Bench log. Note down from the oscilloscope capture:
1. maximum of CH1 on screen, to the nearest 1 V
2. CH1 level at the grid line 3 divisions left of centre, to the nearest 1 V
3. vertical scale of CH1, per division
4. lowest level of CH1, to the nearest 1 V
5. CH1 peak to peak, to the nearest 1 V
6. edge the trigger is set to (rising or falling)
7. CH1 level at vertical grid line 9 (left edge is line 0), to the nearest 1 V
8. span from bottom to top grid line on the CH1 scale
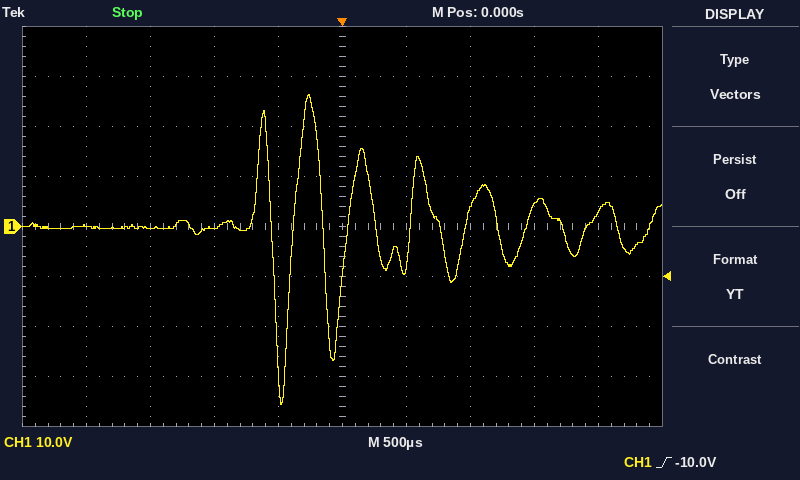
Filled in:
26 V
0 V
10 V
-36 V
62 V
rising
3 V
80 V
